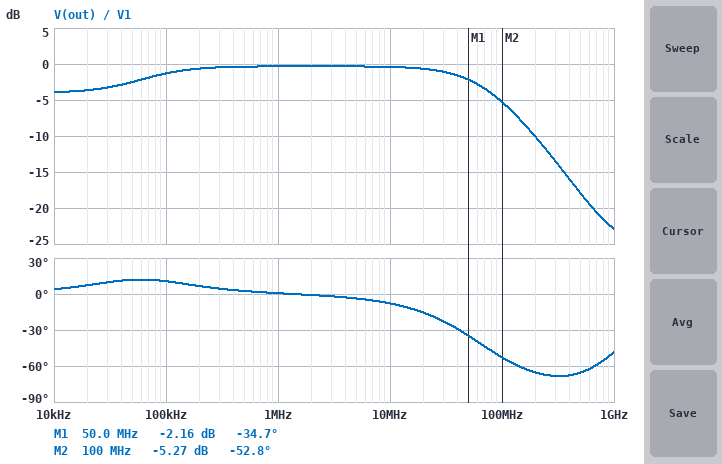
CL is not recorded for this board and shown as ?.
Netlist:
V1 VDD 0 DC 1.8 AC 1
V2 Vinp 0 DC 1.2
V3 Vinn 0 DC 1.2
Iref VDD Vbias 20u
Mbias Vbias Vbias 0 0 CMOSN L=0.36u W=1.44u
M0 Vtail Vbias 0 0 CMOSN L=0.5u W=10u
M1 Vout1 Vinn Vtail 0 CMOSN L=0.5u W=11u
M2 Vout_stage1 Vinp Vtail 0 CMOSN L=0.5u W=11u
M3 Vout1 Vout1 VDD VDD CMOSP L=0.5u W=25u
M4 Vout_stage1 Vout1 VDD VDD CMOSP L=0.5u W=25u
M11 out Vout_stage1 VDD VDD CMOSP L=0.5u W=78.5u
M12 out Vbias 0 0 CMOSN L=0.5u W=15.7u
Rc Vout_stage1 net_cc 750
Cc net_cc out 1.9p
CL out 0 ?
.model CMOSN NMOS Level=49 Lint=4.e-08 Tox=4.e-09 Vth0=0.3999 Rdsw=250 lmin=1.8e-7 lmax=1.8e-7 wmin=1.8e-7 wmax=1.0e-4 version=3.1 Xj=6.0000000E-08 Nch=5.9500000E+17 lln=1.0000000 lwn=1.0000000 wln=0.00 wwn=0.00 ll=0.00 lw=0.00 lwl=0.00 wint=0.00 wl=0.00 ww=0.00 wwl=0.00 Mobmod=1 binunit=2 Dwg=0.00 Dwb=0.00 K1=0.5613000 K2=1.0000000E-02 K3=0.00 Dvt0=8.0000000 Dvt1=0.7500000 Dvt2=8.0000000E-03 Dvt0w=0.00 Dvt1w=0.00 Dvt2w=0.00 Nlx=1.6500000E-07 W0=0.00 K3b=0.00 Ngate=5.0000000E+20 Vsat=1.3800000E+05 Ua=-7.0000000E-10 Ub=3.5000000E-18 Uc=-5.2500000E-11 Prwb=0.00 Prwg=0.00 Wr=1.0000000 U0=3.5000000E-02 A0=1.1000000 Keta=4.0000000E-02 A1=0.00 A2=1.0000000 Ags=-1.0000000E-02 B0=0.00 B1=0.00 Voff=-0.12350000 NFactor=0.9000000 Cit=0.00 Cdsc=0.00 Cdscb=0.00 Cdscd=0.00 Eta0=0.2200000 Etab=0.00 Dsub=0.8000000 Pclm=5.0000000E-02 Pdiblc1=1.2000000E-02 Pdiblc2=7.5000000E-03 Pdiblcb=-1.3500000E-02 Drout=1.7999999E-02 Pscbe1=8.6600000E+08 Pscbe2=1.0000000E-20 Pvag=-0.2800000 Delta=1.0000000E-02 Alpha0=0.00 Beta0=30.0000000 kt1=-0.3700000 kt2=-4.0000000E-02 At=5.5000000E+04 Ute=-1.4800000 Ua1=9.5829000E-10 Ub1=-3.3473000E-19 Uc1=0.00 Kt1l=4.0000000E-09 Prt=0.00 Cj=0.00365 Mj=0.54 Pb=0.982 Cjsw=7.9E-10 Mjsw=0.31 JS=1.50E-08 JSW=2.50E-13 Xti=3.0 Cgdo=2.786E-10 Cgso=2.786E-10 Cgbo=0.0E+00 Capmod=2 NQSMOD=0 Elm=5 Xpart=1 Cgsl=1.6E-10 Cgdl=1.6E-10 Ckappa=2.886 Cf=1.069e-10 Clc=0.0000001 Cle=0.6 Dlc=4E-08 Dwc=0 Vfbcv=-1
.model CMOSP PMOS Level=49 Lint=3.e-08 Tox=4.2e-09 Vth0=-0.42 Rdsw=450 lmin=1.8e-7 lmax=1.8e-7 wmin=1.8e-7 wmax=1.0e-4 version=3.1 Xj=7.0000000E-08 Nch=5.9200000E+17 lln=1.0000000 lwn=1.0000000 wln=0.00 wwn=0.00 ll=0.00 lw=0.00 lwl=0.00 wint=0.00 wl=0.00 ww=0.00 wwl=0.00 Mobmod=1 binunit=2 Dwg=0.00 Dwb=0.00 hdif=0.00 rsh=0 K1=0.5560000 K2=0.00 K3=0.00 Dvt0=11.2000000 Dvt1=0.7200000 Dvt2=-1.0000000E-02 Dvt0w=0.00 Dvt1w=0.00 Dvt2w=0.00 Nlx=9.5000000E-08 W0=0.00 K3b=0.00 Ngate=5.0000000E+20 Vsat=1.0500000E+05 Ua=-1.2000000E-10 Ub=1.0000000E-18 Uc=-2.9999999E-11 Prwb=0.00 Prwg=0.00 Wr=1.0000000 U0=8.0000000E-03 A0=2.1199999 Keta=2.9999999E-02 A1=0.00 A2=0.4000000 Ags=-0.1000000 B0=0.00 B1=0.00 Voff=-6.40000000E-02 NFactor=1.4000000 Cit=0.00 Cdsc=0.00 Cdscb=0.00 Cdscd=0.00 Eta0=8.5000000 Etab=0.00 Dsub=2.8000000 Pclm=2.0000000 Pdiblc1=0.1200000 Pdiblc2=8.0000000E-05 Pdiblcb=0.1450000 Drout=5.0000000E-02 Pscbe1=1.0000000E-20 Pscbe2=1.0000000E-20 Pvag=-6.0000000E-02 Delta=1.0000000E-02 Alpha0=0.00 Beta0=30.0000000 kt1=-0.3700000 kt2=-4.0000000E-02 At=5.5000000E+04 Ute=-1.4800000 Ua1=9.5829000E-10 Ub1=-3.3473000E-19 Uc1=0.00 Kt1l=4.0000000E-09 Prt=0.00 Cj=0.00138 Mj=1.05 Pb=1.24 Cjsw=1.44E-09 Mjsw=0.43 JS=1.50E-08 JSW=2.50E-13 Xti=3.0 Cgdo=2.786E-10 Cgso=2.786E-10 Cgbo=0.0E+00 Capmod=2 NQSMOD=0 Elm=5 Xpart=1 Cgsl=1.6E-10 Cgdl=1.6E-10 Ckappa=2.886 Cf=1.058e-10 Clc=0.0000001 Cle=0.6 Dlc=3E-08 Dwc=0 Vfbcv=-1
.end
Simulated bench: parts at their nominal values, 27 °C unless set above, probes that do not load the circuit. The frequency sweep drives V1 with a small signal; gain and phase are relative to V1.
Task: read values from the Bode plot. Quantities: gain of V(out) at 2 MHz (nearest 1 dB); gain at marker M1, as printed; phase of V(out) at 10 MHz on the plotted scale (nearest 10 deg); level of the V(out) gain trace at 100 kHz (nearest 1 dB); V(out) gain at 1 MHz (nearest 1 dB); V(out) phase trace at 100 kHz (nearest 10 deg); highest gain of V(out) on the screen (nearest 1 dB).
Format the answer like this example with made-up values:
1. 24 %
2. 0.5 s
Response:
1. 0 dB
2. -2.16 dB
3. -10 deg
4. -1 dB
5. 0 dB
6. 10 deg
7. 0 dB
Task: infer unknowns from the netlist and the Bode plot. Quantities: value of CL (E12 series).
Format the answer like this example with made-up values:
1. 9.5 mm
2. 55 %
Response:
1. 3.9 pF
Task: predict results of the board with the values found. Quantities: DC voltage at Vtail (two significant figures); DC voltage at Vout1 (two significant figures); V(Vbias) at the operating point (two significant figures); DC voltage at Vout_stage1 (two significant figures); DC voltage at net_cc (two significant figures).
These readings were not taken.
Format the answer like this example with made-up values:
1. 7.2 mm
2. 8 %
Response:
1. 460 mV
2. 1.1 V
3. 690 mV
4. 1.1 V
5. 1.1 V
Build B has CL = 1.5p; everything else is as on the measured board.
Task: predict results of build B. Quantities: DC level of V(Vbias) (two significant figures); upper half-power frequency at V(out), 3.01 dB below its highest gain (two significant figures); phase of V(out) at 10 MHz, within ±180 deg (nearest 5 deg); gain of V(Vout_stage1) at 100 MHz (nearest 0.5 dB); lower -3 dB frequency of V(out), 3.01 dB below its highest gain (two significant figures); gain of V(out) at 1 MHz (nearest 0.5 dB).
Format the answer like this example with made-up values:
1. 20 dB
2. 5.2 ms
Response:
1. 690 mV
2. 160 MHz
3. -5 deg
4. -2.0 dB
5. 31 kHz
6. 0 dB
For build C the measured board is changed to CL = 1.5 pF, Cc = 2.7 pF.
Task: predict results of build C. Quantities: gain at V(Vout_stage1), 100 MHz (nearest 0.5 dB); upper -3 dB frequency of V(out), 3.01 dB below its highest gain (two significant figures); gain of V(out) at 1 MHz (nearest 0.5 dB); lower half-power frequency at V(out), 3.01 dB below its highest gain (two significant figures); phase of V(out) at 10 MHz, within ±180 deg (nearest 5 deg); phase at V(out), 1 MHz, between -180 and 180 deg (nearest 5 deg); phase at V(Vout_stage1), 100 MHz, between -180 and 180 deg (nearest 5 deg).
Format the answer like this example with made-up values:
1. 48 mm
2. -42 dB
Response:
1. -2.0 dB
2. 170 MHz
3. 0 dB
4. 22 kHz
5. -5 deg
6. 0 deg
7. -25 deg
